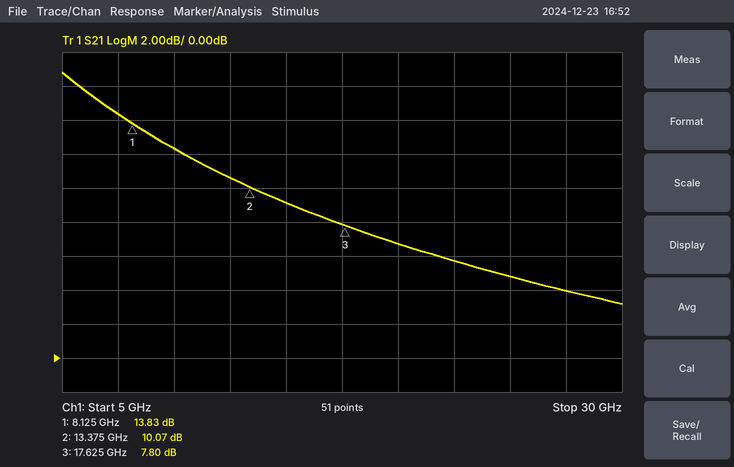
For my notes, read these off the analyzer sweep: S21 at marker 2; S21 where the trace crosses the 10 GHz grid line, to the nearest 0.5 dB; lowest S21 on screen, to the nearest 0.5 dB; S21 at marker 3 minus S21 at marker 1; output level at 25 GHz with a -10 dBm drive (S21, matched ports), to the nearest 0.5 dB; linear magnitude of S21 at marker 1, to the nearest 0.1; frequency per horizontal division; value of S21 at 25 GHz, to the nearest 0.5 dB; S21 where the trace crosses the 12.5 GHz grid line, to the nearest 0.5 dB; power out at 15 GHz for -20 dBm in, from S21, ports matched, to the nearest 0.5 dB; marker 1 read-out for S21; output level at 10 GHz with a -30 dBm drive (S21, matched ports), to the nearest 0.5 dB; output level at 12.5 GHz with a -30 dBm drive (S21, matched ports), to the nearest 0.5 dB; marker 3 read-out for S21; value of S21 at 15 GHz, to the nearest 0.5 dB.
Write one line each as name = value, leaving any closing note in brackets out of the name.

S21 at marker 2 = 10.07 dB
S21 where the trace crosses the 10 GHz grid line, to the nearest 0.5 dB = 12.5 dB
lowest S21 on screen, to the nearest 0.5 dB = 3.0 dB
S21 at marker 3 minus S21 at marker 1 = -6.03 dB
output level at 25 GHz with a -10 dBm drive (S21, matched ports), to the nearest 0.5 dB = -5.0 dBm
linear magnitude of S21 at marker 1, to the nearest 0.1 = 4.9
frequency per horizontal division = 2.5 GHz
value of S21 at 25 GHz, to the nearest 0.5 dB = 5.0 dB
S21 where the trace crosses the 12.5 GHz grid line, to the nearest 0.5 dB = 10.5 dB
power out at 15 GHz for -20 dBm in, from S21, ports matched, to the nearest 0.5 dB = -11.0 dBm
marker 1 read-out for S21 = 13.83 dB
output level at 10 GHz with a -30 dBm drive (S21, matched ports), to the nearest 0.5 dB = -17.5 dBm
output level at 12.5 GHz with a -30 dBm drive (S21, matched ports), to the nearest 0.5 dB = -19.5 dBm
marker 3 read-out for S21 = 7.80 dB
value of S21 at 15 GHz, to the nearest 0.5 dB = 9.0 dB
